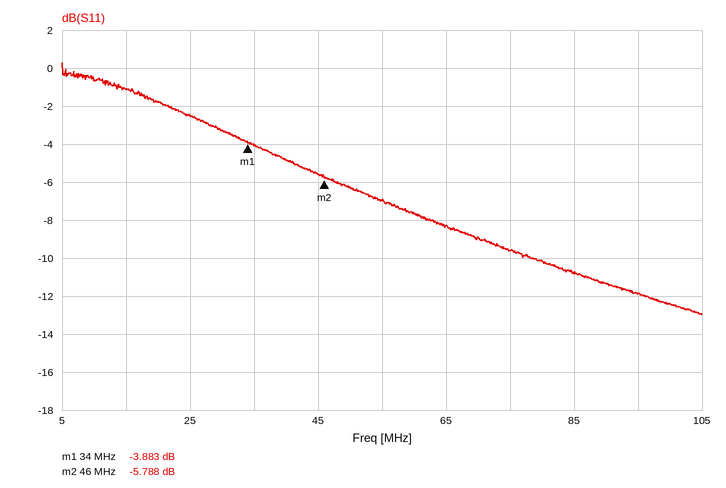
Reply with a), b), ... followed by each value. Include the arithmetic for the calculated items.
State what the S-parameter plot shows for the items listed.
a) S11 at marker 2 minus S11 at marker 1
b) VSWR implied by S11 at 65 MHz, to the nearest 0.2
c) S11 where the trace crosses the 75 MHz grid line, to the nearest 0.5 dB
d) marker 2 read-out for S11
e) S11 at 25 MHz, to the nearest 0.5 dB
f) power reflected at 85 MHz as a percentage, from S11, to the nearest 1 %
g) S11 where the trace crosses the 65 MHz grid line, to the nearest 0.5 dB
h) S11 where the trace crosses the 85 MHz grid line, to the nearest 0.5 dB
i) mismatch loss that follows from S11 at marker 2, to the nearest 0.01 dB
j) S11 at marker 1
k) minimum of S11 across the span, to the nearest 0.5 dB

a) -5.788 − (-3.883) = -1.905 dB
b) |Γ| = 10^(-8.5/20) = 0.3758; VSWR = (1 + 0.3758)/(1 − 0.3758) ≈ 2.2
c) -9.5 dB
d) -5.788 dB
e) -2.5 dB
f) 10^(-11/10) ≈ 8 %
g) -8.5 dB
h) -11.0 dB
i) −10 log10(1 − 10^(-5.788/10)) ≈ 1.33 dB
j) -3.883 dB
k) -13.0 dB
